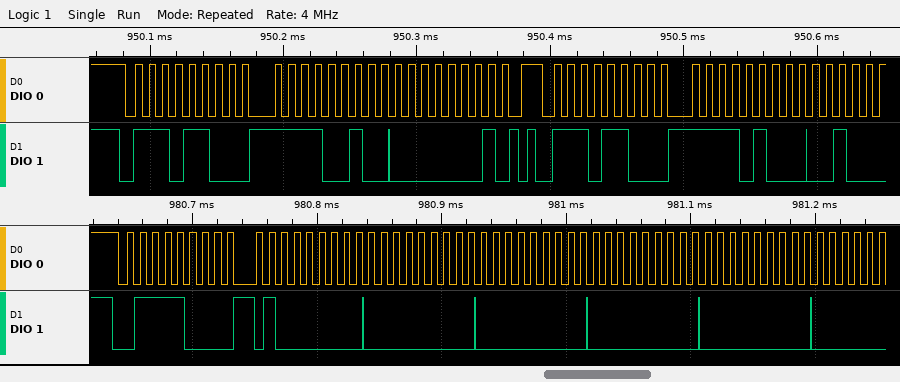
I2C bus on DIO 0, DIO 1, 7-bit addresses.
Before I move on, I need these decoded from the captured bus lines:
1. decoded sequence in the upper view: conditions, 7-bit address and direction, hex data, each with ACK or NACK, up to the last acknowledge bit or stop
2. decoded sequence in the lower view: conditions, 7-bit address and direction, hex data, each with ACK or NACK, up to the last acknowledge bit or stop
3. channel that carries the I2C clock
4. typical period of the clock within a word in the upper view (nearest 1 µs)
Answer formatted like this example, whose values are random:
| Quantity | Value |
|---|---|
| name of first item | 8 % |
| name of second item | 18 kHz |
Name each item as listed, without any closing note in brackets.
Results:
| Quantity | Value |
|---|---|
| decoded sequence in the upper view: conditions, 7-bit address and direction, hex data, each with ACK or NACK, up to the last acknowledge bit or stop | start, address 76 write ACK, F2 ACK, 01 ACK, stop, start, address 76 write ACK, F4 ACK |
| decoded sequence in the lower view: conditions, 7-bit address and direction, hex data, each with ACK or NACK, up to the last acknowledge bit or stop | start, address 3C write ACK, 40 ACK, 00 ACK, 00 ACK, 00 ACK, 00 ACK |
| channel that carries the I2C clock | DIO 0 |
| typical period of the clock within a word in the upper view | 10 µs |
